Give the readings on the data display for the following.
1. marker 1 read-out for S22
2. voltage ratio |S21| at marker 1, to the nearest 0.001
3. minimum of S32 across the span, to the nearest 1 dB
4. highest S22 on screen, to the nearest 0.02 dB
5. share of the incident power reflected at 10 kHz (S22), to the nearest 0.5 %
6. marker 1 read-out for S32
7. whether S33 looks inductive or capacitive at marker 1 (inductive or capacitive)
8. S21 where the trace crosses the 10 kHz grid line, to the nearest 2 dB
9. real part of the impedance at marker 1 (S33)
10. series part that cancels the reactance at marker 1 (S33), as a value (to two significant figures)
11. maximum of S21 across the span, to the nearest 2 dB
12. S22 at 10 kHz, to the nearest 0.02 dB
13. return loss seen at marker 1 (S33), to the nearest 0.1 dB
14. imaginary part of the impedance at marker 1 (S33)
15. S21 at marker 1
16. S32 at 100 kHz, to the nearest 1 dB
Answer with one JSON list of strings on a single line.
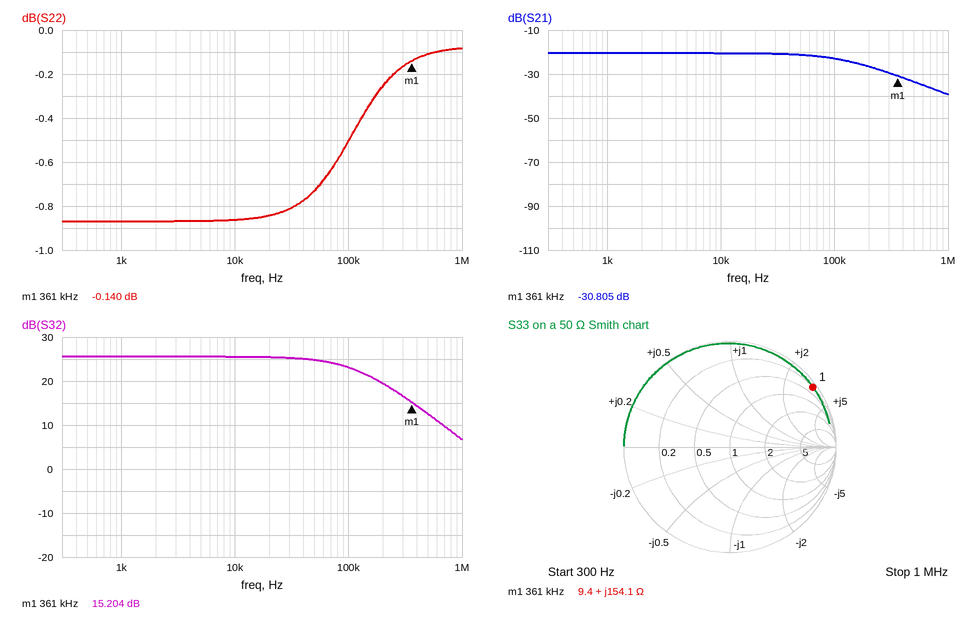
["-0.140 dB", "0.029", "7 dB", "-0.08 dB", "82.0 %", "15.204 dB", "inductive", "-20 dB", "9.4 Ω", "2.9 nF", "-20 dB", "-0.86 dB", "0.3 dB", "+154.1 Ω", "-30.805 dB", "23 dB"]
